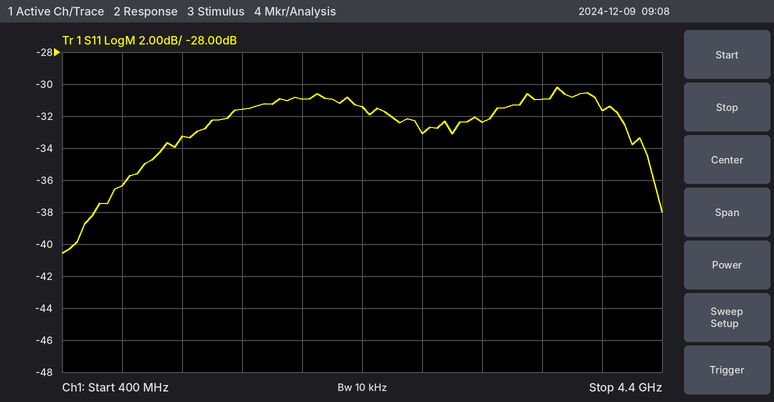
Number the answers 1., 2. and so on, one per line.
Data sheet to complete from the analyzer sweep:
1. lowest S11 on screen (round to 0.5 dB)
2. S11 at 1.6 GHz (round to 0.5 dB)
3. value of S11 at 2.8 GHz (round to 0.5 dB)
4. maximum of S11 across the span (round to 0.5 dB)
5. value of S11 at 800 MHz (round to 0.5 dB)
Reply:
1. -40.5 dB
2. -31.5 dB
3. -33.0 dB
4. -30.0 dB
5. -36.5 dB
